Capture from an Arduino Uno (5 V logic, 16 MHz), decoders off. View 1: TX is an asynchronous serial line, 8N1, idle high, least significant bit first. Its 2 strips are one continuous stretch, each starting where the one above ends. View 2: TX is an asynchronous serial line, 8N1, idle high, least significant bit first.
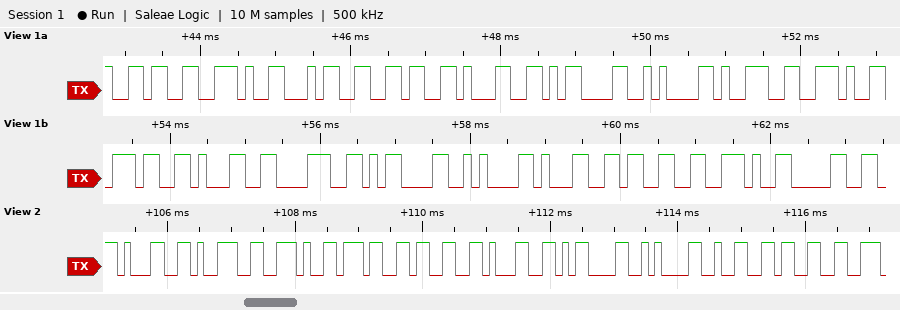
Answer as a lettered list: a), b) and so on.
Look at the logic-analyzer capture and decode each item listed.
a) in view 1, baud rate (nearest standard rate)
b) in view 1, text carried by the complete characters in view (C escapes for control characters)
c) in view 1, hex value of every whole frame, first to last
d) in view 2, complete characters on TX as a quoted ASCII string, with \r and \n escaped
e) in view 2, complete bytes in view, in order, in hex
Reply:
a) 9600 baud
b) "6.461\r\n9.718\r\n13.0"
c) 36 2E 34 36 31 0D 0A 39 2E 37 31 38 0D 0A 31 33 2E 30
d) "19.731\r\n23"
e) 31 39 2E 37 33 31 0D 0A 32 33
